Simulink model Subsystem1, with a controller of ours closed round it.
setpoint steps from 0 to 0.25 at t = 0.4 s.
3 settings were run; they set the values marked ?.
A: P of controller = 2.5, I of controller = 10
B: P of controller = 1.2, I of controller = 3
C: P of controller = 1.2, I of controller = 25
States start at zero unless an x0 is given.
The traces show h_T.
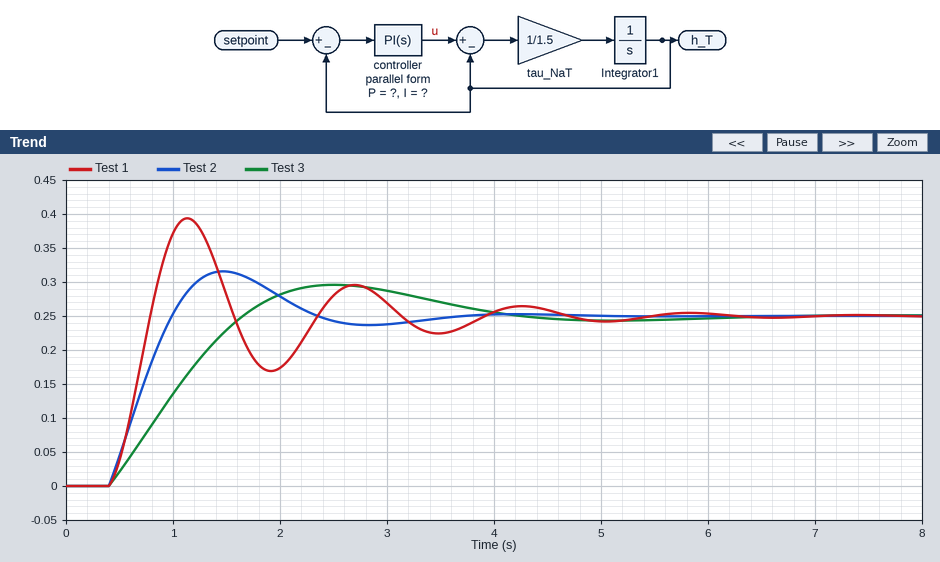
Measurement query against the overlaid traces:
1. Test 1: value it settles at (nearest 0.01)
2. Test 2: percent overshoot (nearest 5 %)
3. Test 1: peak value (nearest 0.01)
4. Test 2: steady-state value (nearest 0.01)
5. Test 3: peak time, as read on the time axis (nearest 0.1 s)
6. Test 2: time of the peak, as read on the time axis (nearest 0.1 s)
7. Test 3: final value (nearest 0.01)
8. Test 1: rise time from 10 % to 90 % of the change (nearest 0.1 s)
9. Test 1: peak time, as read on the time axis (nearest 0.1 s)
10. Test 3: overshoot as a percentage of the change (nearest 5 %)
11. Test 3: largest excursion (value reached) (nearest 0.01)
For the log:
0.25
25 %
0.39
0.25
2.5 s
1.5 s
0.25
0.3 s
1.1 s
20 %
0.30
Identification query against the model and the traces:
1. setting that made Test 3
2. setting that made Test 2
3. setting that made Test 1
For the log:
B
A
C
